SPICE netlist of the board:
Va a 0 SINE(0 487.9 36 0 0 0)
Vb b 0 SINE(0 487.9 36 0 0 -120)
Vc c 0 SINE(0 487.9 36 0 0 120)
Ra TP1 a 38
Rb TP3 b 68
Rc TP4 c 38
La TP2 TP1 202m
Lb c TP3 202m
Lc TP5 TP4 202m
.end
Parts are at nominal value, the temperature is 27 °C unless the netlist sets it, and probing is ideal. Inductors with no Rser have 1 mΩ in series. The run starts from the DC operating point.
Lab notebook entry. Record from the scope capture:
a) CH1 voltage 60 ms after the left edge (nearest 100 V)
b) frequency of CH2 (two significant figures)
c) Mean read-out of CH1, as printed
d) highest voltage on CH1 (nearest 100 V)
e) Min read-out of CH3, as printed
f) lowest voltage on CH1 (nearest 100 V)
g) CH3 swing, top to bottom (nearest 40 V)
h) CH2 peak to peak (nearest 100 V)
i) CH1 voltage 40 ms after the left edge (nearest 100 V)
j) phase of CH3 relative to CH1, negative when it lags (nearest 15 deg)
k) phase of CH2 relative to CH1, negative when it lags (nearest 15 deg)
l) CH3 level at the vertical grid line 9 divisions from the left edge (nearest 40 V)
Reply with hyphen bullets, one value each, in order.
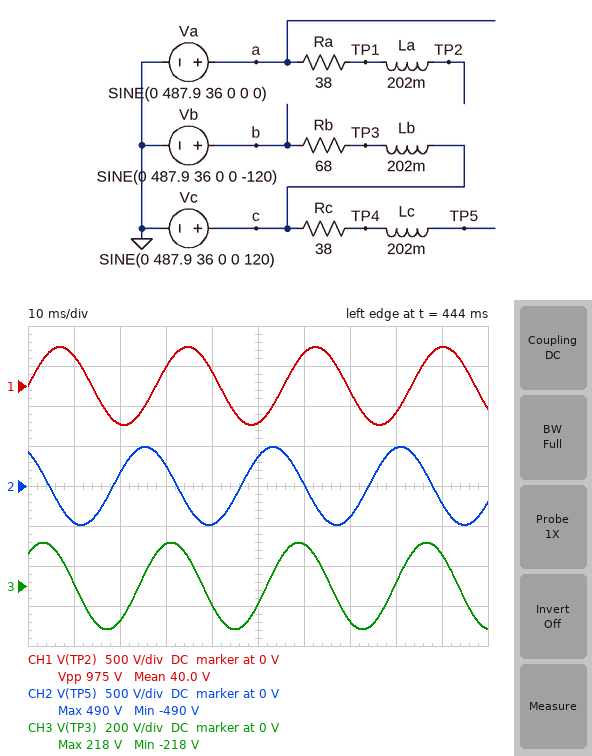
- 400 V
- 36 Hz
- 40.0 V
- 500 V
- -218 V
- -500 V
- 440 V
- 1.0 kV
- 200 V
- 45 deg
- 120 deg
- 160 V
